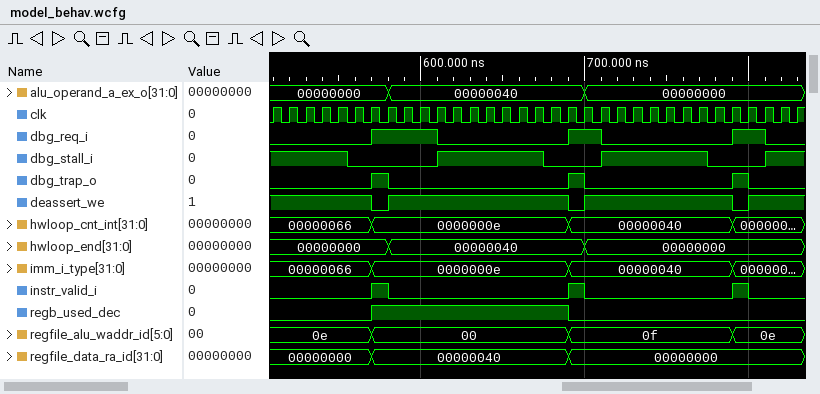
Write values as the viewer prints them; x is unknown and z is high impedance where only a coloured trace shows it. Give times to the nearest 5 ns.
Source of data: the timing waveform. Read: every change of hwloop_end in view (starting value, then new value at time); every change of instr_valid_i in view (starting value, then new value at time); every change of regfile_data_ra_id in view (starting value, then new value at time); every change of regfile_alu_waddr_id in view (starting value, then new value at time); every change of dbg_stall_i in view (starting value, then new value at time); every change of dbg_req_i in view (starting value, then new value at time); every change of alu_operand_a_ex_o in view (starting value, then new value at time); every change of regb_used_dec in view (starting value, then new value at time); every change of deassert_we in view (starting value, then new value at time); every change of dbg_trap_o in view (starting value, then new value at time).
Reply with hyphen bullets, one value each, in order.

- 00000000, 00000040 at 580 ns, 00000000 at 700 ns
- 0, 1 at 570 ns, 0 at 580 ns, 1 at 690 ns, 0 at 700 ns, 1 at 790 ns, 0 at 800 ns
- 00000000, 00000040 at 570 ns, 00000000 at 690 ns
- 0e, 00 at 570 ns, 0f at 690 ns, 0e at 790 ns
- 1, 0 at 555 ns, 1 at 610 ns, 0 at 675 ns, 1 at 710 ns, 0 at 775 ns, 1 at 810 ns
- 0, 1 at 570 ns, 0 at 610 ns, 1 at 690 ns, 0 at 710 ns, 1 at 790 ns, 0 at 810 ns
- 00000000, 00000040 at 580 ns, 00000000 at 700 ns
- 0, 1 at 570 ns, 0 at 690 ns
- 1, 0 at 570 ns, 1 at 580 ns, 0 at 690 ns, 1 at 700 ns, 0 at 790 ns, 1 at 800 ns
- 0, 1 at 570 ns, 0 at 580 ns, 1 at 690 ns, 0 at 700 ns, 1 at 790 ns, 0 at 800 ns
